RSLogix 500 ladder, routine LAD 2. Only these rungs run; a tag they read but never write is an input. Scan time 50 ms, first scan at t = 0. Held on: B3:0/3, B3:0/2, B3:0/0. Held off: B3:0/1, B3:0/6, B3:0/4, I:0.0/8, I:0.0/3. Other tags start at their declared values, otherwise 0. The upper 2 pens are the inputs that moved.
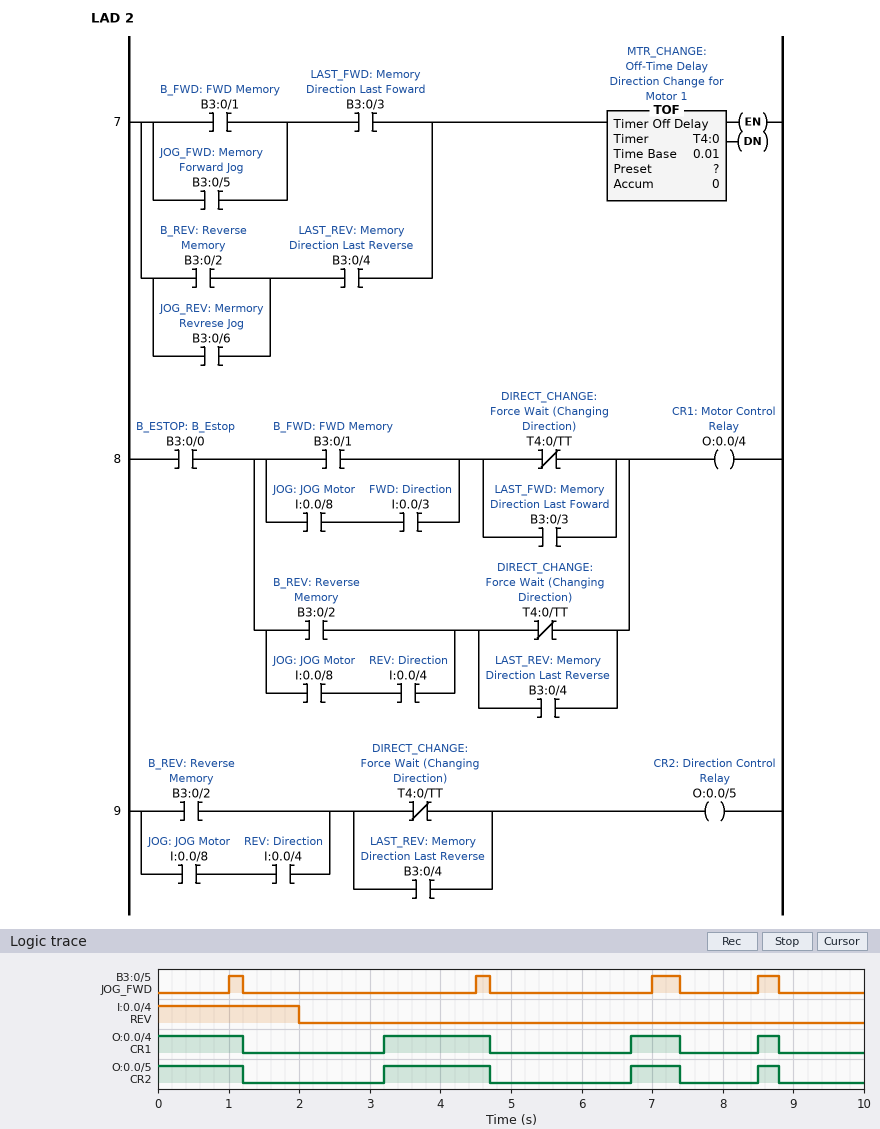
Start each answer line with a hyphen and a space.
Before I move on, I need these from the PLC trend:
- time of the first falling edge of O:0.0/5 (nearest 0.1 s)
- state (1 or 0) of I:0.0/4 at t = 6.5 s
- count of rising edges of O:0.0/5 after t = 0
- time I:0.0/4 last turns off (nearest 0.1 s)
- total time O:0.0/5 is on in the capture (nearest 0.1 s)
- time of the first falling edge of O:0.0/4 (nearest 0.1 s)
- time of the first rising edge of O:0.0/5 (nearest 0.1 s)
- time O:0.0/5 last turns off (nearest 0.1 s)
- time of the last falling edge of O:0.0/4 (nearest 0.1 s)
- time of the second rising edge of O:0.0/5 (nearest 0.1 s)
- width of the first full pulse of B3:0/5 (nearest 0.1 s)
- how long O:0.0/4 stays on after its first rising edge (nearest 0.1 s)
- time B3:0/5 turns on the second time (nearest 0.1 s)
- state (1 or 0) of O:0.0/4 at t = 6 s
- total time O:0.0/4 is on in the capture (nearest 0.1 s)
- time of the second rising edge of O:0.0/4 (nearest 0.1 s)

- 1.2 s
- 0
- 3
- 2.0 s
- 3.7 s
- 1.2 s
- 3.2 s
- 8.8 s
- 8.8 s
- 6.7 s
- 0.2 s
- 1.5 s
- 4.5 s
- 0
- 3.7 s
- 6.7 s
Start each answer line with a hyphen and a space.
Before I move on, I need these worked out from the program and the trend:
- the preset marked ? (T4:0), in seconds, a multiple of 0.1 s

- 2.0 s
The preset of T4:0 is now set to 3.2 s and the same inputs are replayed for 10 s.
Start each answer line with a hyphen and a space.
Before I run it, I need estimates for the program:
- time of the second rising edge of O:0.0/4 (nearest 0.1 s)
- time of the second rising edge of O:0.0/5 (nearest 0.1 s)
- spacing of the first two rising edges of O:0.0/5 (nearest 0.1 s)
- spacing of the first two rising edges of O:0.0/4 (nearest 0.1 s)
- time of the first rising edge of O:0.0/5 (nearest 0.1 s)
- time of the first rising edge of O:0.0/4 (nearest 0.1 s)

- 7.0 s
- 7.0 s
- 2.6 s
- 2.6 s
- 4.4 s
- 4.4 s
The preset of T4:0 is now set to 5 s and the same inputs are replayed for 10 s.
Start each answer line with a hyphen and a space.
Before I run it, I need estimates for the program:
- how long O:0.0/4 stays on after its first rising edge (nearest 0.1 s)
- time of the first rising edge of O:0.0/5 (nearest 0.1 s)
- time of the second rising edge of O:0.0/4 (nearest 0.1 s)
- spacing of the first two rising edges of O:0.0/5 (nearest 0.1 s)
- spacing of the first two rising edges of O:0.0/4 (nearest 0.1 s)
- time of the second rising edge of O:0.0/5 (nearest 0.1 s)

- 0.2 s
- 4.5 s
- 7.0 s
- 2.5 s
- 2.5 s
- 7.0 s
